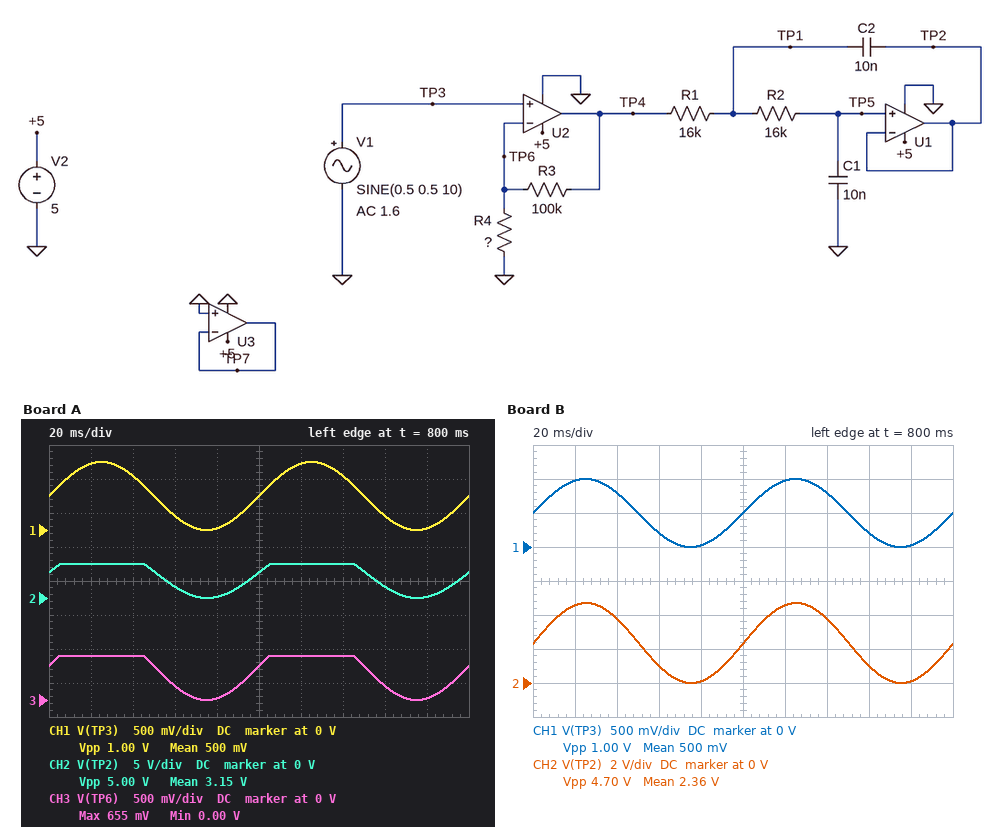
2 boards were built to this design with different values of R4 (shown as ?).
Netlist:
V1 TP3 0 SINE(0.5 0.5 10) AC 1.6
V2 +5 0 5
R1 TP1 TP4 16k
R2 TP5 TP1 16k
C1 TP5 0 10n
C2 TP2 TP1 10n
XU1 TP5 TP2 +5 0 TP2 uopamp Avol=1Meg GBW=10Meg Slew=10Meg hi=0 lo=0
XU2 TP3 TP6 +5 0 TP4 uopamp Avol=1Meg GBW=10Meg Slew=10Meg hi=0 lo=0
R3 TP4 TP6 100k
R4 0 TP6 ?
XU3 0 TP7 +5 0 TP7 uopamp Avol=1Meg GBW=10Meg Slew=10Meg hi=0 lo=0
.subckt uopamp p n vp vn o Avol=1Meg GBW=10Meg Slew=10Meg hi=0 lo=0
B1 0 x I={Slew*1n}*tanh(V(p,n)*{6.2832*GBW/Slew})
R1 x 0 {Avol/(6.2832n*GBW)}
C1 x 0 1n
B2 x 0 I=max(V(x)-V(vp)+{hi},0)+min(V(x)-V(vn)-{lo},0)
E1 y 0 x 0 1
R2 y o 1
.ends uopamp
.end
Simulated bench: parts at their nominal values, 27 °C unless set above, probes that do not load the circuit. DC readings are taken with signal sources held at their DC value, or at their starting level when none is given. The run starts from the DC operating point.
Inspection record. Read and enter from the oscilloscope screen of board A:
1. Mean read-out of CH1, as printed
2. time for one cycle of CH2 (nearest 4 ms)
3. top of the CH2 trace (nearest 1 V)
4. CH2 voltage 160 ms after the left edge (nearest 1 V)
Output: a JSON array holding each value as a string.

["500 mV", "100 ms", "5 V", "2 V"]
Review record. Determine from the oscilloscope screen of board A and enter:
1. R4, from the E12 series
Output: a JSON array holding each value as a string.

["15 kΩ"]
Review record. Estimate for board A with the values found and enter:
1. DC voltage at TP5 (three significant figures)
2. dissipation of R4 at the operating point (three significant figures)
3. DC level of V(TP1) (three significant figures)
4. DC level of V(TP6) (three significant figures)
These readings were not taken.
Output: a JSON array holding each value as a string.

["3.83 V", "16.7 µW", "3.83 V", "500 mV"]
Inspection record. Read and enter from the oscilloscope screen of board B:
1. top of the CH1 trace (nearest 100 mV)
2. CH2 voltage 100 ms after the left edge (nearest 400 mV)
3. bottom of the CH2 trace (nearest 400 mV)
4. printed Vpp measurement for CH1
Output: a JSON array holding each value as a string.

["1.0 V", "2.4 V", "0 V", "1.00 V"]
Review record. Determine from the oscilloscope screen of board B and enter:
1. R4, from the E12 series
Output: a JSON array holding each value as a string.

["27 kΩ"]
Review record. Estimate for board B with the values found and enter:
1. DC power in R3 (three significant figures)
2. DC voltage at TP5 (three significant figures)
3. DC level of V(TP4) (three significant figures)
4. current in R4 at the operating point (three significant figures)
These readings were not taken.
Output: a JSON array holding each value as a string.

["34.3 µW", "2.35 V", "2.35 V", "18.5 µA"]
